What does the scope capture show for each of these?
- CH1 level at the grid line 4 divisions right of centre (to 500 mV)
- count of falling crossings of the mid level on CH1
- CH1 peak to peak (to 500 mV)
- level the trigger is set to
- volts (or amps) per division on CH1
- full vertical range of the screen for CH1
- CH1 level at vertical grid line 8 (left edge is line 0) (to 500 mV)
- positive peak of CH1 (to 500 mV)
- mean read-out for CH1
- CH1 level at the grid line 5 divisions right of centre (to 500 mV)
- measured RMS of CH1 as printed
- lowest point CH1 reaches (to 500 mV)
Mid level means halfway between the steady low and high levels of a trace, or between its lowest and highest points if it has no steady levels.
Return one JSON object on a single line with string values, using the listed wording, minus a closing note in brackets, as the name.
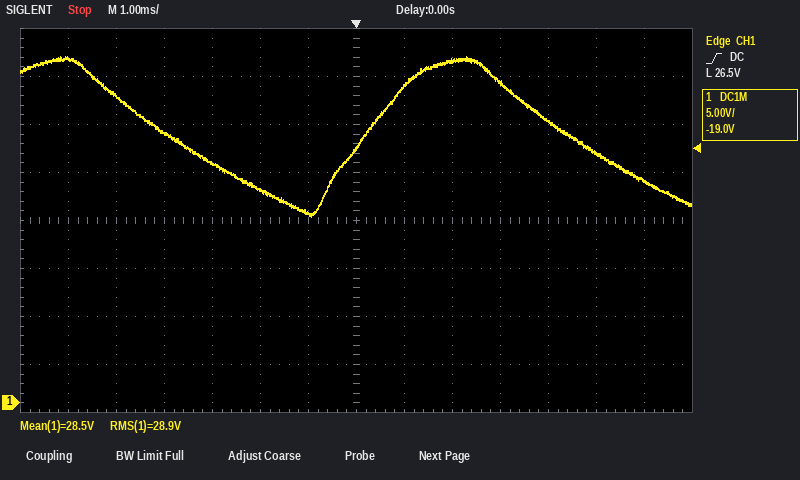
{"CH1 level at the grid line 4 divisions right of centre": "29.5 V", "count of falling crossings of the mid level on CH1": "2", "CH1 peak to peak": "16.5 V", "level the trigger is set to": "26.5 V", "volts (or amps) per division on CH1": "5 V", "full vertical range of the screen for CH1": "40 V", "CH1 level at vertical grid line 8 (left edge is line 0)": "33.0 V", "positive peak of CH1": "36.0 V", "mean read-out for CH1": "28.5 V", "CH1 level at the grid line 5 divisions right of centre": "26.0 V", "measured RMS of CH1 as printed": "28.9 V", "lowest point CH1 reaches": "19.5 V"}
